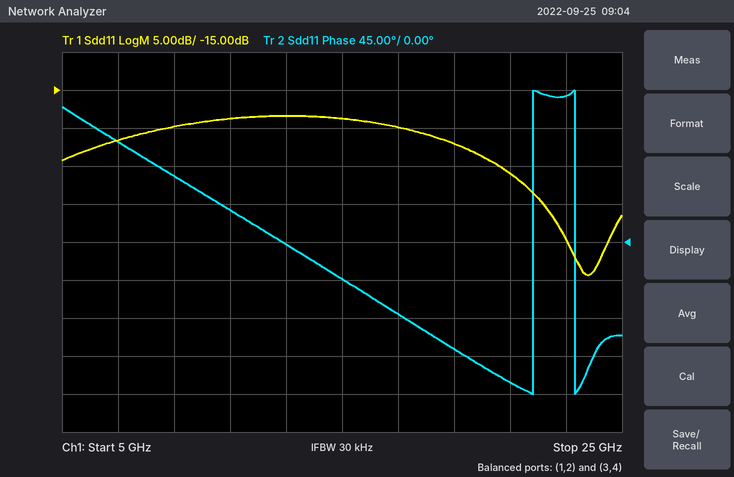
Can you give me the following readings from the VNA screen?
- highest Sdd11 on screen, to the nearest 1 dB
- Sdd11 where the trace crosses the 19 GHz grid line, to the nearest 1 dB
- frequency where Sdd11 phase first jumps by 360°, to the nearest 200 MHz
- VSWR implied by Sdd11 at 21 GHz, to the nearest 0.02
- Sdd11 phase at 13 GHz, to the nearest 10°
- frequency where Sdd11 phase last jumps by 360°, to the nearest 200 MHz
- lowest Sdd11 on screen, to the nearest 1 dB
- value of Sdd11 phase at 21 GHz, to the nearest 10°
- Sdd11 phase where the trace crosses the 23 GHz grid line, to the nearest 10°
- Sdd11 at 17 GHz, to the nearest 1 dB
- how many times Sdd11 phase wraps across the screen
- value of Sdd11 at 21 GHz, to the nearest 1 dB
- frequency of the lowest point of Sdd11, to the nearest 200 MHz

-18 dB
-22 dB
21.8 GHz
1.10
0°
23.4 GHz
-39 dB
-170°
170°
-20 dB
2
-26 dB
23.8 GHz
